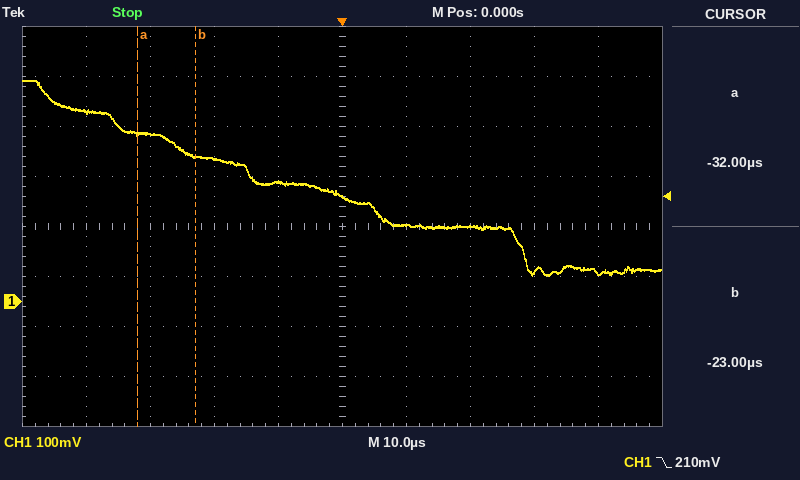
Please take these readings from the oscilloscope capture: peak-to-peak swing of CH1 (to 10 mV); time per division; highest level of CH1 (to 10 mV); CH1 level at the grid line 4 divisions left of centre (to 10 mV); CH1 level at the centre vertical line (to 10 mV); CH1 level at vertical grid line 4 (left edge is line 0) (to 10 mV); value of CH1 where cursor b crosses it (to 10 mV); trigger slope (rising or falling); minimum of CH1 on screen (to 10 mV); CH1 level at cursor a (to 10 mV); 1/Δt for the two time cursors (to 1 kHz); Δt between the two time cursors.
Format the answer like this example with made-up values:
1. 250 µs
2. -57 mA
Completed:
1. 390 mV
2. 10 µs
3. 440 mV
4. 380 mV
5. 210 mV
6. 240 mV
7. 290 mV
8. falling
9. 50 mV
10. 340 mV
11. 111 kHz
12. 9 µs
